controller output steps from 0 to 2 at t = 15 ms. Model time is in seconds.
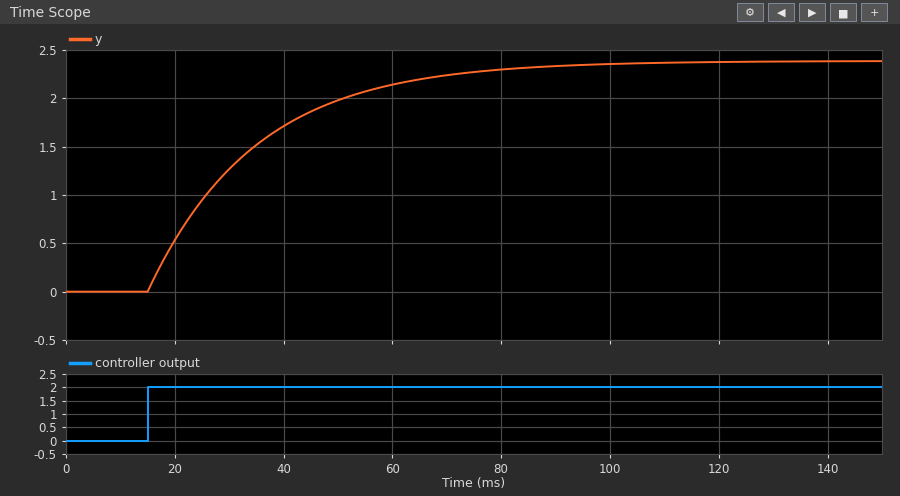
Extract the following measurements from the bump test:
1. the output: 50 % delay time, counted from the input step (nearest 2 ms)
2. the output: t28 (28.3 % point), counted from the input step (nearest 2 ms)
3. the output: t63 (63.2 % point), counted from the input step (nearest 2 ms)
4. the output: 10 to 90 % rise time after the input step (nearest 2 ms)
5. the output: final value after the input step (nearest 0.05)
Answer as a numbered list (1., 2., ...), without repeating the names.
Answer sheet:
1. 14 ms
2. 6 ms
3. 20 ms
4. 44 ms
5. 2.40
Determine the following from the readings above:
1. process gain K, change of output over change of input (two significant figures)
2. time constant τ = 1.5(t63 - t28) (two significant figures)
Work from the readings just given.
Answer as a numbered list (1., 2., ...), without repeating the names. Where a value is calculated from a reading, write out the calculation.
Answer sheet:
1. (2.4 - 0) / 2 = 1.2
2. 1.5 × (20 - 6) = 21 ms
